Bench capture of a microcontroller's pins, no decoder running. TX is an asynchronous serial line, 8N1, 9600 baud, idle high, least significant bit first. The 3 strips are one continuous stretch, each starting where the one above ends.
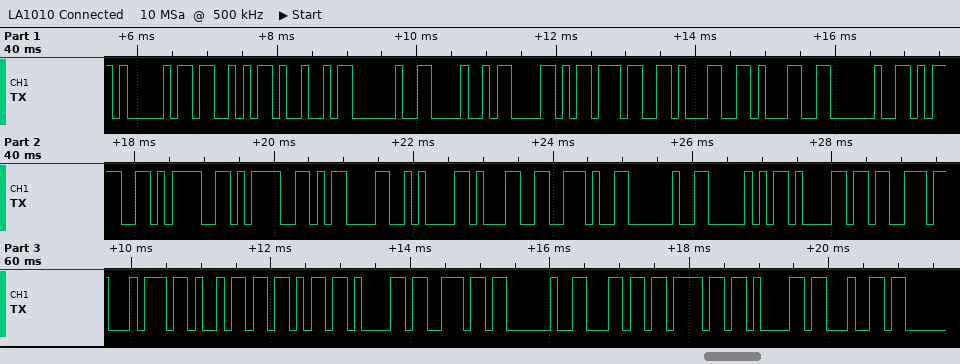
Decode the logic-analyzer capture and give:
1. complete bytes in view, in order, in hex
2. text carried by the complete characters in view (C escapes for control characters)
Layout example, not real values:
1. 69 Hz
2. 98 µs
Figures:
1. 41 53 49 20 48 58 37 31 31 20 3D 3D 3D 0D 0A 31 2E 20 50 61 73 74 69 6B 61 6E 20 6C 6F 61 64
2. "ASI HX711 ===\r\n1. Pastikan load"
